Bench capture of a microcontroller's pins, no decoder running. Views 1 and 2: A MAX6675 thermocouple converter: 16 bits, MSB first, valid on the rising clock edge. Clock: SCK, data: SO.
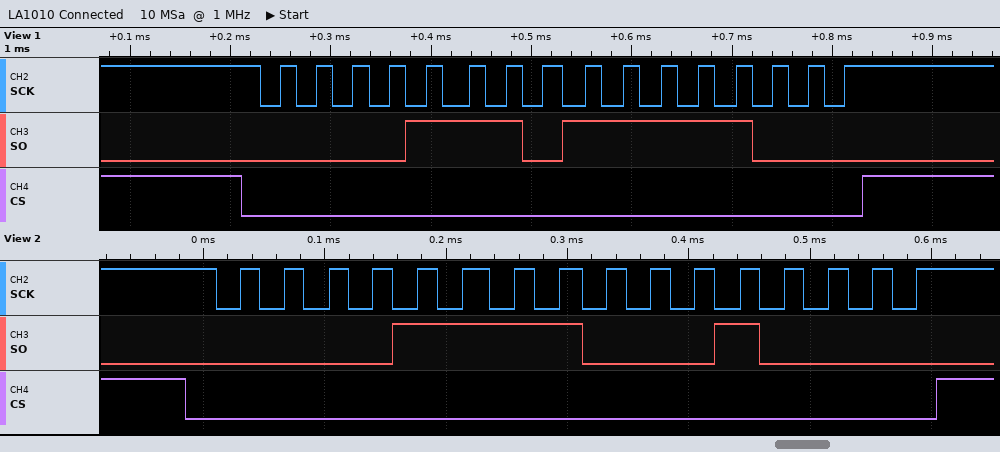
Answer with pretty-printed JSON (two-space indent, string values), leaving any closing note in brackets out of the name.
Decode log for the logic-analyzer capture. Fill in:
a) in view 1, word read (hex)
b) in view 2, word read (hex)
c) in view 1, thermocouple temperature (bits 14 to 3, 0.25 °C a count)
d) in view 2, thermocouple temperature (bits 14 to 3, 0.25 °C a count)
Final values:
{
  "in view 1, word read": "0x0EF8",
  "in view 2, word read": "0x0F10",
  "in view 1, thermocouple temperature": "119.75 °C",
  "in view 2, thermocouple temperature": "120.50 °C"
}
